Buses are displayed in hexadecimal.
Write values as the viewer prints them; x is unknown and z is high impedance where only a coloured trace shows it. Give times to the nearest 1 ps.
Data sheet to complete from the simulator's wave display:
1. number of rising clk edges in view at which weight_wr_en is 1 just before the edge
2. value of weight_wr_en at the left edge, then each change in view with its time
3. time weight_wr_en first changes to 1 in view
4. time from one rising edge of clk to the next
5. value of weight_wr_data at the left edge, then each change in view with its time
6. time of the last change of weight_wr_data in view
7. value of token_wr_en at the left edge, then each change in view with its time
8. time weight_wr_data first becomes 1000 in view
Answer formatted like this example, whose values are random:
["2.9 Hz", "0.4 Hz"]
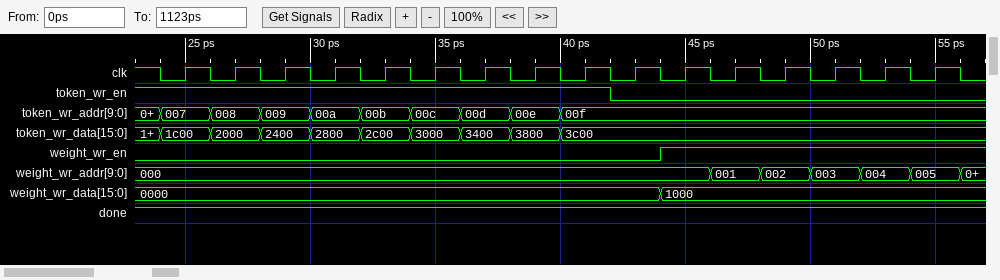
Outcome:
["6", "0, 1 at 44 ps", "44 ps", "2 ps", "0000, 1000 at 44 ps", "44 ps", "1, 0 at 42 ps", "44 ps"]
